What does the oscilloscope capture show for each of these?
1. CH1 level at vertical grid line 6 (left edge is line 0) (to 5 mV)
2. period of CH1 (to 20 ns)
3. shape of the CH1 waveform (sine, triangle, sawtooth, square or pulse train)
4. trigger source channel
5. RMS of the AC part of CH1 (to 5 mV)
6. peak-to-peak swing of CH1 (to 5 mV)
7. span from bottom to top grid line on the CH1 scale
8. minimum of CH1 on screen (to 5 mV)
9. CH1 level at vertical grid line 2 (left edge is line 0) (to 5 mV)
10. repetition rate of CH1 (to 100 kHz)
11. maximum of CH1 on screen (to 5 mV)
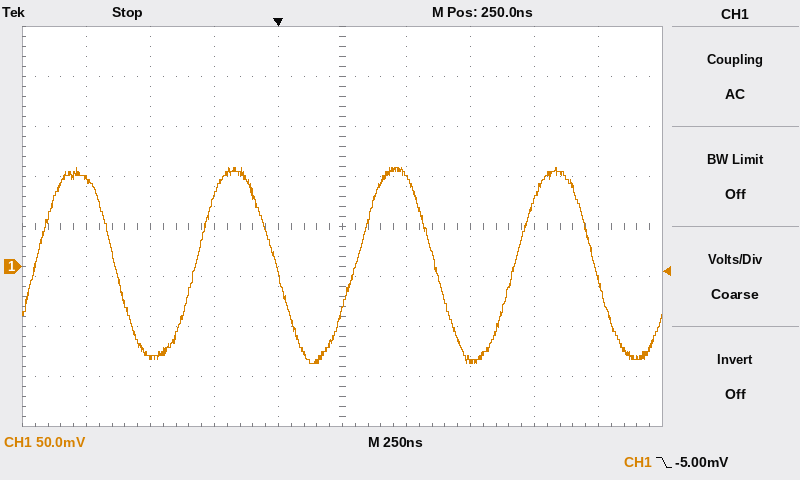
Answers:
90 mV
620 ns
sine
CH1
70 mV
195 mV
400 mV
-95 mV
-90 mV
1.6 MHz
100 mV
